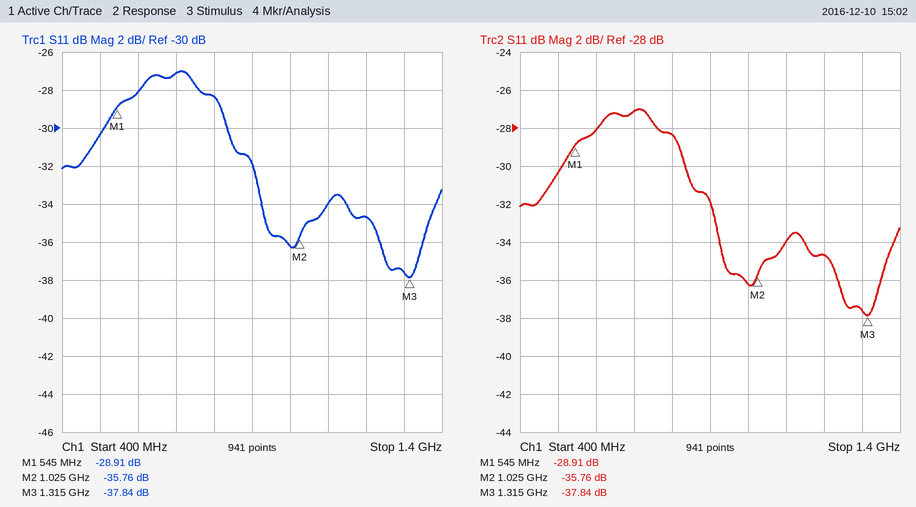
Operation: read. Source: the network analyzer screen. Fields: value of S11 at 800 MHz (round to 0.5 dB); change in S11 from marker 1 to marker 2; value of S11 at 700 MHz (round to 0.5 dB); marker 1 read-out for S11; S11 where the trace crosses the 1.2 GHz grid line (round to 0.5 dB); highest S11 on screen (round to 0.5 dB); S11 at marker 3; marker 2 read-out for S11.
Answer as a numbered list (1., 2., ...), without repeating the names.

1. -28.5 dB
2. -6.85 dB
3. -27.0 dB
4. -28.91 dB
5. -34.5 dB
6. -27.0 dB
7. -37.84 dB
8. -35.76 dB
